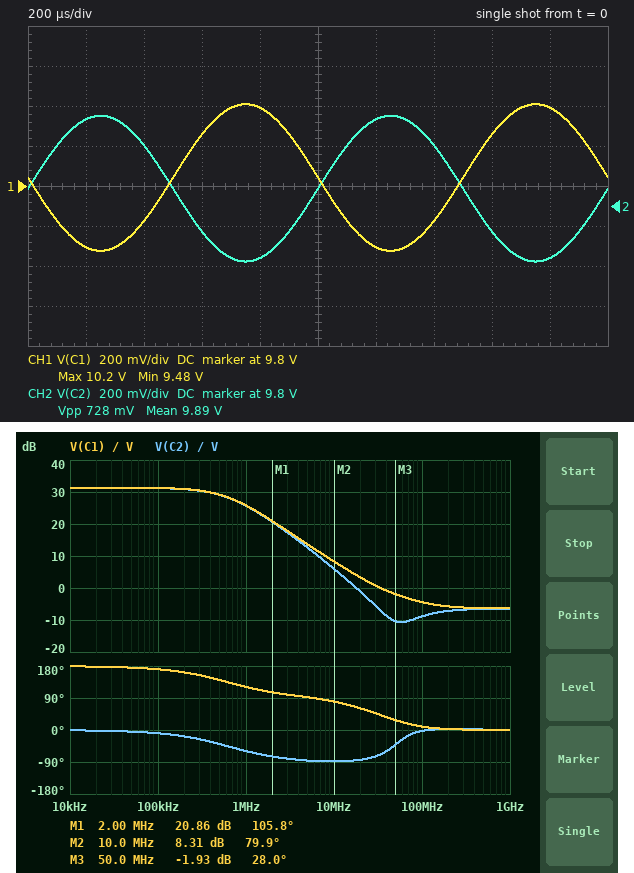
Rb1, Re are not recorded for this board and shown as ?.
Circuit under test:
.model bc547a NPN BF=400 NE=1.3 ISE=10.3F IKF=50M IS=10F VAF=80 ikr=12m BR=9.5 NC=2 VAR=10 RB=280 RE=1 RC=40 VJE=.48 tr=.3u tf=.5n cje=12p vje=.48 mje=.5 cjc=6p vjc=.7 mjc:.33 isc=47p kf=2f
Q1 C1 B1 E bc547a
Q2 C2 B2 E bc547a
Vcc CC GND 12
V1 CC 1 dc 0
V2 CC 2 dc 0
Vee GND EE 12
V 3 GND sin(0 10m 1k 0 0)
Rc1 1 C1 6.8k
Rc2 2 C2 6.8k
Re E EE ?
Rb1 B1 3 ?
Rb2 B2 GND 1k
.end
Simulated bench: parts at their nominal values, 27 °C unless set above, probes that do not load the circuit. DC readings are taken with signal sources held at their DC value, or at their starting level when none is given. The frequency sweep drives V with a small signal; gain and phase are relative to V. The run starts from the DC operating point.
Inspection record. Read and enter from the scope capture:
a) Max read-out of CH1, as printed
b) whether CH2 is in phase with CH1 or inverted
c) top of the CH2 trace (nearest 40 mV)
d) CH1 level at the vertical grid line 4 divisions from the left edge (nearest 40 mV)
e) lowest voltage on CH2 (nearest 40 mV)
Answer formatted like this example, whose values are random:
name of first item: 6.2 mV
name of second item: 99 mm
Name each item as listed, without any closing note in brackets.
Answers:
Max read-out of CH1, as printed: 10.2 V
whether CH2 is in phase with CH1 or inverted: inverted
top of the CH2 trace: 10.24 V
CH1 level at the vertical grid line 4 divisions from the left edge: 10.20 V
lowest voltage on CH2: 9.52 V
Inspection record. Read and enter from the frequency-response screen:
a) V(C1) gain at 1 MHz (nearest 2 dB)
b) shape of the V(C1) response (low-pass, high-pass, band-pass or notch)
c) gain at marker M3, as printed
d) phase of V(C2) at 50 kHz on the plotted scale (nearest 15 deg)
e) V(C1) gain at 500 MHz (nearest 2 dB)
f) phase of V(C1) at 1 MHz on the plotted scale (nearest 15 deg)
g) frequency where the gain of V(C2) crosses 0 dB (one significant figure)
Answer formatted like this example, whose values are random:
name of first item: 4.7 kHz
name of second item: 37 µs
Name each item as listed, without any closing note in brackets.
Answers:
V(C1) gain at 1 MHz: 26 dB
shape of the V(C1) response: low-pass
gain at marker M3, as printed: -1.93 dB
phase of V(C2) at 50 kHz on the plotted scale: 0 deg
V(C1) gain at 500 MHz: -6 dB
phase of V(C1) at 1 MHz on the plotted scale: 120 deg
frequency where the gain of V(C2) crosses 0 dB: 20 MHz
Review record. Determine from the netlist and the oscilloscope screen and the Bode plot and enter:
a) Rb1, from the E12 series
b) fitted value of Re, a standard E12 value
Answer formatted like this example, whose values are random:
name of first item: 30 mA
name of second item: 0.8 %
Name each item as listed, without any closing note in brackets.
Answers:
Rb1, from the E12 series: 680 Ω
fitted value of Re, a standard E12 value: 18 kΩ
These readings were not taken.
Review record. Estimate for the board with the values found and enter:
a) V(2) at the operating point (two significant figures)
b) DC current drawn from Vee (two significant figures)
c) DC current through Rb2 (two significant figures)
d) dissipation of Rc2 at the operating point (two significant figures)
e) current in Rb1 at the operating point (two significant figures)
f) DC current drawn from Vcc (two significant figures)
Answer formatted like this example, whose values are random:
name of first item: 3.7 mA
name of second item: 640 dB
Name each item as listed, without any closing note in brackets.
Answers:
V(2) at the operating point: 12 V
DC current drawn from Vee: 630 µA
DC current through Rb2: 1.9 µA
dissipation of Rc2 at the operating point: 660 µW
current in Rb1 at the operating point: 1.9 µA
DC current drawn from Vcc: 630 µA
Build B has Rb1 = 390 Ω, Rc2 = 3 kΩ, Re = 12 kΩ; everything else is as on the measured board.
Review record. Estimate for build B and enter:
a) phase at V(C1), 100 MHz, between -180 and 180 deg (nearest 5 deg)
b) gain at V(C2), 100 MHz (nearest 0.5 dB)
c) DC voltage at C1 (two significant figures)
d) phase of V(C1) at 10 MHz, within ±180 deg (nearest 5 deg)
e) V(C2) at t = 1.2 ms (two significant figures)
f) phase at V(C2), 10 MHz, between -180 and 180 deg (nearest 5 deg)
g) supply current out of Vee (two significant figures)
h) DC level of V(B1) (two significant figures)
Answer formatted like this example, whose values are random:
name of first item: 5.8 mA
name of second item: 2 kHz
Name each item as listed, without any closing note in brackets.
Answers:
phase at V(C1), 100 MHz, between -180 and 180 deg: 15 deg
gain at V(C2), 100 MHz: -9.0 dB
DC voltage at C1: 8.7 V
phase of V(C1) at 10 MHz, within ±180 deg: 75 deg
V(C2) at t = 1.2 ms: 11 V
phase at V(C2), 10 MHz, between -180 and 180 deg: -75 deg
supply current out of Vee: 950 µA
DC level of V(B1): -1.1 mV
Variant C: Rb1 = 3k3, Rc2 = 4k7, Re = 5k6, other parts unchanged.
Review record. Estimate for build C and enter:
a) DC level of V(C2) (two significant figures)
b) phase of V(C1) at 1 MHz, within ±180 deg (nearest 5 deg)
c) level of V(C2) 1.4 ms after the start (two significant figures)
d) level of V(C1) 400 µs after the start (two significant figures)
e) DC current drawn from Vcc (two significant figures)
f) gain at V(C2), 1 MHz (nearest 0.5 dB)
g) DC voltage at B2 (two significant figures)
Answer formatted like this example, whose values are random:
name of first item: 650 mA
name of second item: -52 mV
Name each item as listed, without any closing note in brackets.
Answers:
DC level of V(C2): 6.5 V
phase of V(C1) at 1 MHz, within ±180 deg: 95 deg
level of V(C2) 1.4 ms after the start: 6.8 V
level of V(C1) 400 µs after the start: 5.8 V
DC current drawn from Vcc: 2.0 mA
gain at V(C2), 1 MHz: 18.0 dB
DC voltage at B2: -6.3 mV
